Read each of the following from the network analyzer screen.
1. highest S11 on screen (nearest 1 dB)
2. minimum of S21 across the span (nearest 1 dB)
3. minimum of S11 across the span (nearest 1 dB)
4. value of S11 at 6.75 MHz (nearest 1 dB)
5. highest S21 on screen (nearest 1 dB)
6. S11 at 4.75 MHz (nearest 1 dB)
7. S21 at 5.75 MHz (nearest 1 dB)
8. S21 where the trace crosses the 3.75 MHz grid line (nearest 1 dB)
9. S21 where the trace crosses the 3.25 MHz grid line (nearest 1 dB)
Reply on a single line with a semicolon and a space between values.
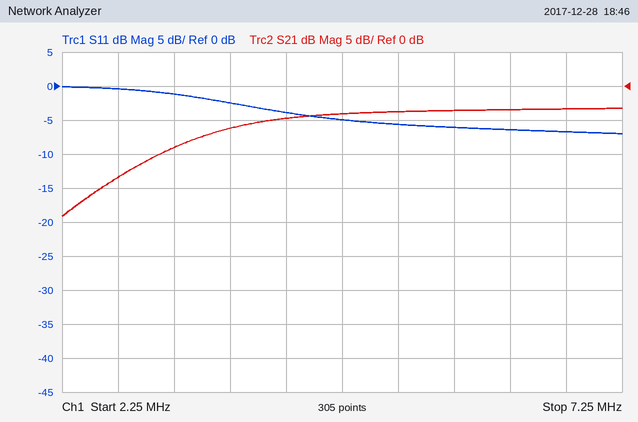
0 dB; -19 dB; -7 dB; -7 dB; -3 dB; -5 dB; -4 dB; -6 dB; -9 dB
